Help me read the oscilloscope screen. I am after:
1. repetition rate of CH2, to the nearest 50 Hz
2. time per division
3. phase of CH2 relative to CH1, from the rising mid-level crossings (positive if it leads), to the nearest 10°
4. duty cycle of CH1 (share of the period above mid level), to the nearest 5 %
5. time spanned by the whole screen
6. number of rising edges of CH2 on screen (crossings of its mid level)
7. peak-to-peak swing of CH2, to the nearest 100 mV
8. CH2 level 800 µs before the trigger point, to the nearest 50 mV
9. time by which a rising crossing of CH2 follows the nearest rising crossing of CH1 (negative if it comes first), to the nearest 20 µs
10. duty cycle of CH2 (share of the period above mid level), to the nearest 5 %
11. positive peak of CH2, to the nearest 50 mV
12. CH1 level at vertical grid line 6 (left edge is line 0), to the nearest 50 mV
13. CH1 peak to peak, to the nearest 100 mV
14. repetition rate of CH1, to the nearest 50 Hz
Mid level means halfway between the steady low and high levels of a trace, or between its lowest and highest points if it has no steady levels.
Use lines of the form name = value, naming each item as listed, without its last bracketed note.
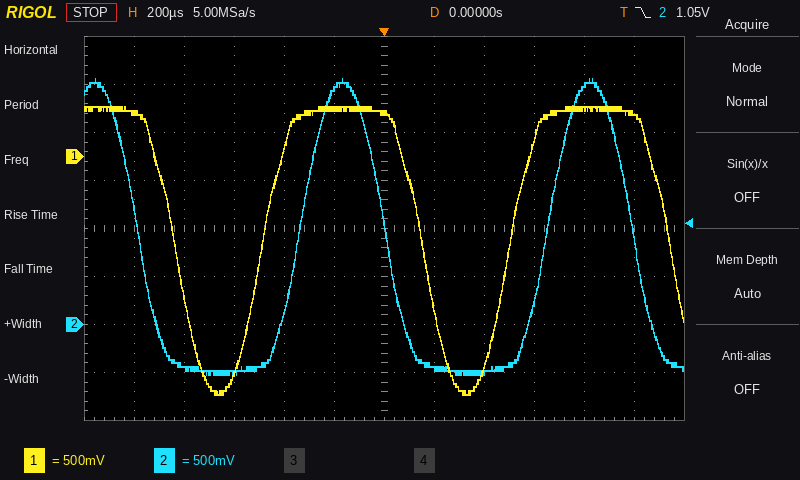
repetition rate of CH2, to the nearest 50 Hz = 1.00 kHz
time per division = 200 µs
phase of CH2 relative to CH1, from the rising mid-level crossings (positive if it leads), to the nearest 10° = -60°
duty cycle of CH1 (share of the period above mid level), to the nearest 5 % = 65 %
time spanned by the whole screen = 2.4 ms
number of rising edges of CH2 on screen = 2
peak-to-peak swing of CH2, to the nearest 100 mV = 3.10 V
CH2 level 800 µs before the trigger point, to the nearest 50 mV = -450 mV
time by which a rising crossing of CH2 follows the nearest rising crossing of CH1 (negative if it comes first), to the nearest 20 µs = +160 µs
duty cycle of CH2 (share of the period above mid level), to the nearest 5 % = 35 %
positive peak of CH2, to the nearest 50 mV = 2.55 V
CH1 level at vertical grid line 6 (left edge is line 0), to the nearest 50 mV = 450 mV
CH1 peak to peak, to the nearest 100 mV = 3.00 V
repetition rate of CH1, to the nearest 50 Hz = 1.00 kHz
